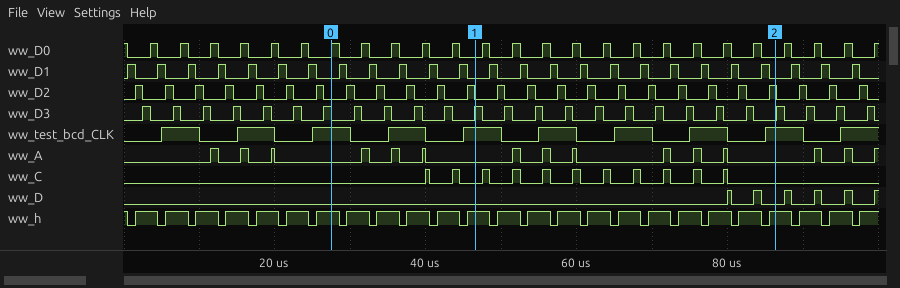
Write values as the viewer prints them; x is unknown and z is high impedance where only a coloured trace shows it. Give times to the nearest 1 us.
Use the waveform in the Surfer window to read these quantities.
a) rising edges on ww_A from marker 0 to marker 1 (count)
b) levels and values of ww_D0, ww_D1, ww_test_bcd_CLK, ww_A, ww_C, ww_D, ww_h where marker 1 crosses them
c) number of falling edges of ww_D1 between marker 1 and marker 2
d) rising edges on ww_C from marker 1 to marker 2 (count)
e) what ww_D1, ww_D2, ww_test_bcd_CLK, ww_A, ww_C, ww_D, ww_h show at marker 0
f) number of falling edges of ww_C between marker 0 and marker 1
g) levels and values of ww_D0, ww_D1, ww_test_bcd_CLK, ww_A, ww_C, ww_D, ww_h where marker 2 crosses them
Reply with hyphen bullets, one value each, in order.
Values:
- 3
- ww_D0=0, ww_D1=0, ww_test_bcd_CLK=1, ww_A=0, ww_C=0, ww_D=0, ww_h=1
- 10
- 9
- ww_D1=0, ww_D2=0, ww_test_bcd_CLK=1, ww_A=0, ww_C=0, ww_D=0, ww_h=1
- 2
- ww_D0=0, ww_D1=0, ww_test_bcd_CLK=1, ww_A=0, ww_C=0, ww_D=0, ww_h=1
